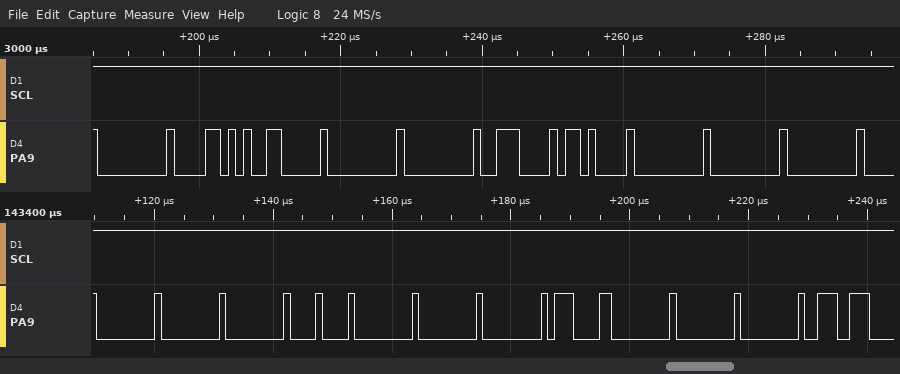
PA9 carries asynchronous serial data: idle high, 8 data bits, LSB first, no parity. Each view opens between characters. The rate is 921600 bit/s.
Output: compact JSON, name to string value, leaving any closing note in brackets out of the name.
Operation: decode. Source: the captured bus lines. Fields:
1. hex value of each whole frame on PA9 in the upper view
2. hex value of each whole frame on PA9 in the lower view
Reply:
{"hex value of each whole frame on PA9 in the upper view": "00, 58, 06, 00, 00, 0E, 0B, 00, 00, 00", "hex value of each whole frame on PA9 in the lower view": "00, 00, 00, 08, 00, 00, 00, 87, 00, 00, 00, CE"}
